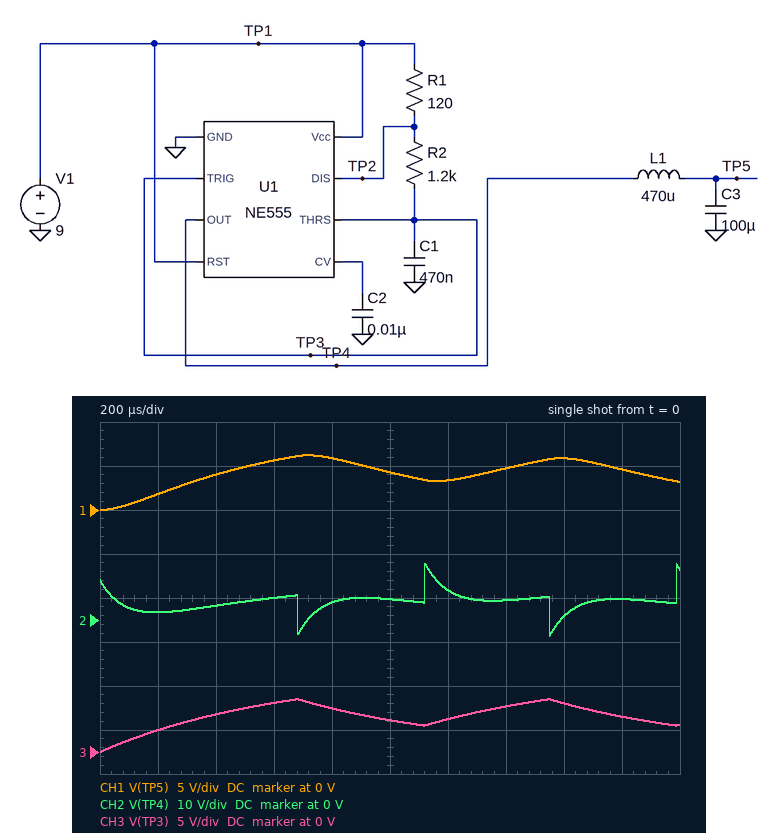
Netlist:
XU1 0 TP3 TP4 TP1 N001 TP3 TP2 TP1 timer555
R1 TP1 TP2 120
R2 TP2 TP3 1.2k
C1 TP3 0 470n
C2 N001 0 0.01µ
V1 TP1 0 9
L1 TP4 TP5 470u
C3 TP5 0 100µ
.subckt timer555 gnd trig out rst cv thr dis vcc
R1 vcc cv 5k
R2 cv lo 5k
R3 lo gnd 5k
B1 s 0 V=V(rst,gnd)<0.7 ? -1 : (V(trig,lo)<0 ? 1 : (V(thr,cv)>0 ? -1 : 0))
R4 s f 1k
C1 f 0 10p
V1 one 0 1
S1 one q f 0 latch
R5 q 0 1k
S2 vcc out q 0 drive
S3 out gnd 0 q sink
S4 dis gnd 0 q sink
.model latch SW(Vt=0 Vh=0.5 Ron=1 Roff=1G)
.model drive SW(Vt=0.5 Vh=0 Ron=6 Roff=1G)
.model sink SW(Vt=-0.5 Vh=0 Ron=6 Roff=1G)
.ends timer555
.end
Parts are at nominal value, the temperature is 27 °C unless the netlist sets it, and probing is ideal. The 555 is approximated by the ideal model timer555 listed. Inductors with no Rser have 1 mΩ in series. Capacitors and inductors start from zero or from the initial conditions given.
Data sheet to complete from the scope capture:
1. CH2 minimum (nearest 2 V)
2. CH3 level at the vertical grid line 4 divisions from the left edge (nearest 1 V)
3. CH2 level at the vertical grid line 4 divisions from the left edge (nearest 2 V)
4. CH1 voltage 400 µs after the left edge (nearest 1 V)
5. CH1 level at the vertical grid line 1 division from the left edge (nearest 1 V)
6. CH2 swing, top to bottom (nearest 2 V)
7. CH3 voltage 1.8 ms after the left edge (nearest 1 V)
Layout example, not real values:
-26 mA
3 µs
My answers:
-4 V
5 V
4 V
4 V
2 V
16 V
4 V
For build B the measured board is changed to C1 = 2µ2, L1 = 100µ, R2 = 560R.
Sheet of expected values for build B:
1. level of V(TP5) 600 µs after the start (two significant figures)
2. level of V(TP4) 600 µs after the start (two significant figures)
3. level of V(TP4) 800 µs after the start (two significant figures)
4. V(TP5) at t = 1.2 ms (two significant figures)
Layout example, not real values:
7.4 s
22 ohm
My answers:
5.7 V
5.6 V
6.6 V
7.8 V
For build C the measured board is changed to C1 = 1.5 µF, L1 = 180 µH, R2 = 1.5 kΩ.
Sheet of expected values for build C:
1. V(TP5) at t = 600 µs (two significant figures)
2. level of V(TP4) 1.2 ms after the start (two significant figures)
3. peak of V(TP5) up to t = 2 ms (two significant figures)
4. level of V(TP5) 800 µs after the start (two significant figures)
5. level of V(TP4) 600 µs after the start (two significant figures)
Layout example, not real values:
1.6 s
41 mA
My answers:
5.7 V
7.8 V
8.7 V
6.7 V
5.5 V
